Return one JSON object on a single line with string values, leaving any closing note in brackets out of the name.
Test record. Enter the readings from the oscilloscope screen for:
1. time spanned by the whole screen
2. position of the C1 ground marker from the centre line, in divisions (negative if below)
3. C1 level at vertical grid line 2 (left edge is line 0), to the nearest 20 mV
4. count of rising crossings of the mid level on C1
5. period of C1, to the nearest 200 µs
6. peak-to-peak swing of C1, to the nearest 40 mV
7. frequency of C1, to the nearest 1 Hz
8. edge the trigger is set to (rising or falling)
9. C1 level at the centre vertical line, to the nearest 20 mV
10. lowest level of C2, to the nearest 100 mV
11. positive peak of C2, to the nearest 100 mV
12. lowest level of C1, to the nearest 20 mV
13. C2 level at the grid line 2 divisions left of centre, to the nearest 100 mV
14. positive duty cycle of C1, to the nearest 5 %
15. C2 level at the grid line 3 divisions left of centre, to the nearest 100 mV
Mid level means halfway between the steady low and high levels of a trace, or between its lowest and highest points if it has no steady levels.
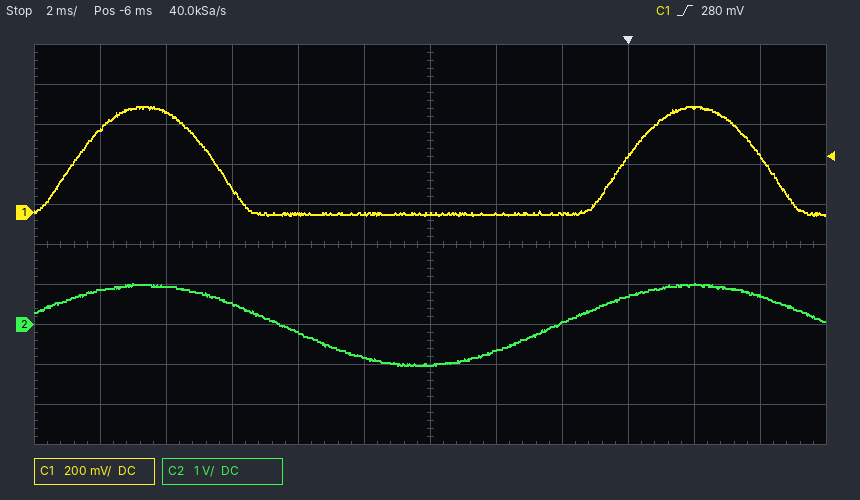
{"time spanned by the whole screen": "24 ms", "position of the C1 ground marker from the centre line, in divisions": "+0.8 div", "C1 level at vertical grid line 2 (left edge is line 0), to the nearest 20 mV": "500 mV", "count of rising crossings of the mid level on C1": "2", "period of C1, to the nearest 200 µs": "16.6 ms", "peak-to-peak swing of C1, to the nearest 40 mV": "560 mV", "frequency of C1, to the nearest 1 Hz": "60 Hz", "edge the trigger is set to": "rising", "C1 level at the centre vertical line, to the nearest 20 mV": "0 mV", "lowest level of C2, to the nearest 100 mV": "-1.0 V", "positive peak of C2, to the nearest 100 mV": "1.0 V", "lowest level of C1, to the nearest 20 mV": "-20 mV", "C2 level at the grid line 2 divisions left of centre, to the nearest 100 mV": "-200 mV", "positive duty cycle of C1, to the nearest 5 %": "25 %", "C2 level at the grid line 3 divisions left of centre, to the nearest 100 mV": "500 mV"}
